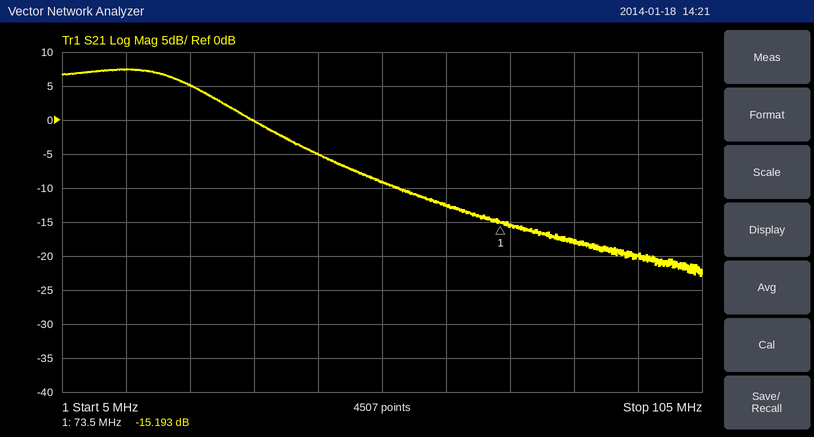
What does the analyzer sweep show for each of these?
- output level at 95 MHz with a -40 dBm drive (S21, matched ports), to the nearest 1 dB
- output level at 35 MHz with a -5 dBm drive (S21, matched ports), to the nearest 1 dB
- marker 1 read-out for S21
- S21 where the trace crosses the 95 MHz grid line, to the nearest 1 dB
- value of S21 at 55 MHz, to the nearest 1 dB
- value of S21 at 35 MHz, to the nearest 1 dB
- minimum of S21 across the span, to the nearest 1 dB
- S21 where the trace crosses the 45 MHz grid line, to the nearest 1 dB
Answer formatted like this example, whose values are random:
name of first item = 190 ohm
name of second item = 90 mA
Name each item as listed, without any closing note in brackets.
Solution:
output level at 95 MHz with a -40 dBm drive (S21, matched ports), to the nearest 1 dB = -60 dBm
output level at 35 MHz with a -5 dBm drive (S21, matched ports), to the nearest 1 dB = -5 dBm
marker 1 read-out for S21 = -15.193 dB
S21 where the trace crosses the 95 MHz grid line, to the nearest 1 dB = -20 dB
value of S21 at 55 MHz, to the nearest 1 dB = -9 dB
value of S21 at 35 MHz, to the nearest 1 dB = 0 dB
minimum of S21 across the span, to the nearest 1 dB = -23 dB
S21 where the trace crosses the 45 MHz grid line, to the nearest 1 dB = -5 dB
